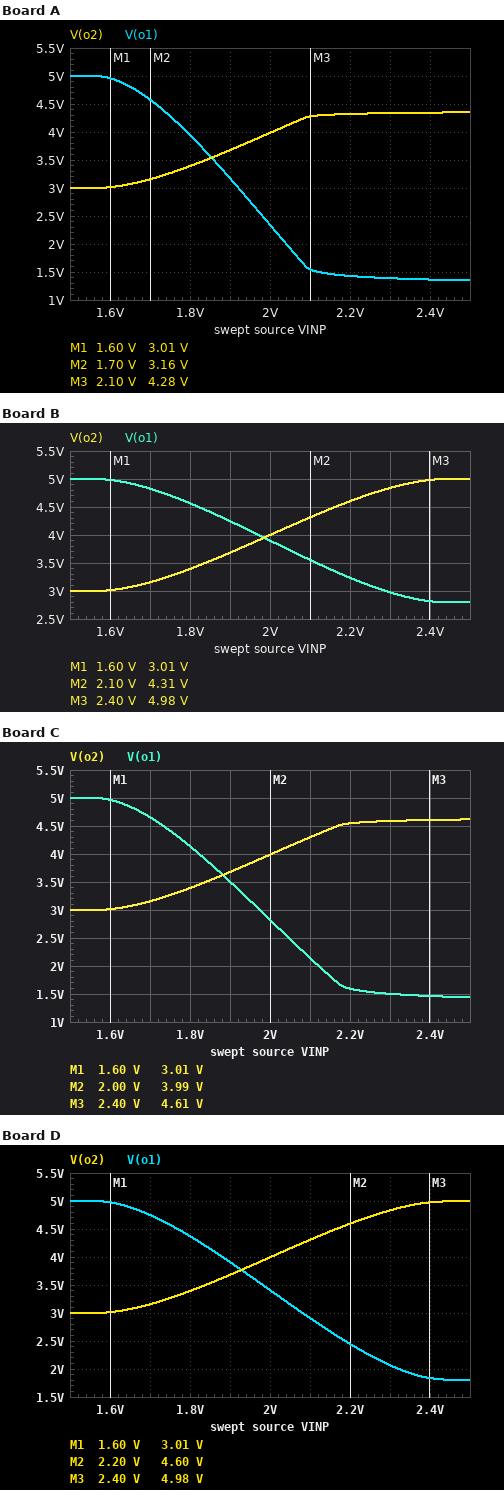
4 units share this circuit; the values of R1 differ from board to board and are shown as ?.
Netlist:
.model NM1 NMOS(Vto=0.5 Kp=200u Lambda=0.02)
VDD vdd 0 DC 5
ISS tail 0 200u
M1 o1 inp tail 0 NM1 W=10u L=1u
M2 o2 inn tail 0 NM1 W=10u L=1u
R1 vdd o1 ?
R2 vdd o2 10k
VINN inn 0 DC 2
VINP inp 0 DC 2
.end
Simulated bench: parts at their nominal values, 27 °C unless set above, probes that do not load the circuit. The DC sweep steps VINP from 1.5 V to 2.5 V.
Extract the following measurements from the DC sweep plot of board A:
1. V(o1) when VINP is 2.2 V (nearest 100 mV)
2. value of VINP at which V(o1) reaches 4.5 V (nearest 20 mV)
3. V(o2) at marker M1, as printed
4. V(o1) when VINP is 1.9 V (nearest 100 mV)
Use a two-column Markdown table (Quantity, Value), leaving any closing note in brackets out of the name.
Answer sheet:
| Quantity | Value |
|---|---|
| V(o1) when VINP is 2.2 V | 1.4 V |
| value of VINP at which V(o1) reaches 4.5 V | 1.72 V |
| V(o2) at marker M1, as printed | 3.01 V |
| V(o1) when VINP is 1.9 V | 3.2 V |
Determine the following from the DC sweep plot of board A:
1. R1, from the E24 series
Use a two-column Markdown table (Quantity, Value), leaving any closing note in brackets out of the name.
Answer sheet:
| Quantity | Value |
|---|---|
| R1, from the E24 series | 27 kΩ |
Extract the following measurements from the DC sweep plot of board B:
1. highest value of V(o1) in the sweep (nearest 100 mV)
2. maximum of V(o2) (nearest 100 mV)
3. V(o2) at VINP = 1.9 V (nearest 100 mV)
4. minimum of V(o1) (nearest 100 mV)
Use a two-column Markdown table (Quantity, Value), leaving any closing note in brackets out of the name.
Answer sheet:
| Quantity | Value |
|---|---|
| highest value of V(o1) in the sweep | 5.0 V |
| maximum of V(o2) | 5.0 V |
| V(o2) at VINP = 1.9 V | 3.7 V |
| minimum of V(o1) | 2.8 V |
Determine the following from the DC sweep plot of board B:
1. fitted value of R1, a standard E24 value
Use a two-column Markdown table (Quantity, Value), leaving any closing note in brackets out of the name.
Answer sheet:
| Quantity | Value |
|---|---|
| fitted value of R1, a standard E24 value | 11 kΩ |
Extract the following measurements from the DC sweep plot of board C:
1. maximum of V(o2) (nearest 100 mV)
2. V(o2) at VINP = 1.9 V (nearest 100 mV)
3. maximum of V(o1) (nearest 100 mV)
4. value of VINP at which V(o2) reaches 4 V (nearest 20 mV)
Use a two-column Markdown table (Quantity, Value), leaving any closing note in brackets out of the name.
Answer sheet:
| Quantity | Value |
|---|---|
| maximum of V(o2) | 4.6 V |
| V(o2) at VINP = 1.9 V | 3.7 V |
| maximum of V(o1) | 5.0 V |
| value of VINP at which V(o2) reaches 4 V | 2.00 V |
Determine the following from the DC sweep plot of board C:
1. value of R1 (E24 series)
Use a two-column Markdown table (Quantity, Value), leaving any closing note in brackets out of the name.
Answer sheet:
| Quantity | Value |
|---|---|
| value of R1 | 22 kΩ |
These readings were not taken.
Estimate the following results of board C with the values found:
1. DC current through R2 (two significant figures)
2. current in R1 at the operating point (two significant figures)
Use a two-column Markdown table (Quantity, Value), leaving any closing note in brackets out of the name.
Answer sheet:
| Quantity | Value |
|---|---|
| DC current through R2 | 100 µA |
| current in R1 at the operating point | 99 µA |
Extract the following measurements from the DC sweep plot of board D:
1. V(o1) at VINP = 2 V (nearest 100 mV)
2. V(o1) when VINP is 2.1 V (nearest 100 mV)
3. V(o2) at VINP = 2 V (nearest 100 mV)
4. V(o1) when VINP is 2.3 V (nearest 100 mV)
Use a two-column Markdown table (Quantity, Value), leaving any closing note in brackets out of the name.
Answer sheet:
| Quantity | Value |
|---|---|
| V(o1) at VINP = 2 V | 3.4 V |
| V(o1) when VINP is 2.1 V | 2.9 V |
| V(o2) at VINP = 2 V | 4.0 V |
| V(o1) when VINP is 2.3 V | 2.1 V |
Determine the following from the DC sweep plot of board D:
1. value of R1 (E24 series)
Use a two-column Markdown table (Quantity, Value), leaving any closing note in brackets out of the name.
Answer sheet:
| Quantity | Value |
|---|---|
| value of R1 | 16 kΩ |
